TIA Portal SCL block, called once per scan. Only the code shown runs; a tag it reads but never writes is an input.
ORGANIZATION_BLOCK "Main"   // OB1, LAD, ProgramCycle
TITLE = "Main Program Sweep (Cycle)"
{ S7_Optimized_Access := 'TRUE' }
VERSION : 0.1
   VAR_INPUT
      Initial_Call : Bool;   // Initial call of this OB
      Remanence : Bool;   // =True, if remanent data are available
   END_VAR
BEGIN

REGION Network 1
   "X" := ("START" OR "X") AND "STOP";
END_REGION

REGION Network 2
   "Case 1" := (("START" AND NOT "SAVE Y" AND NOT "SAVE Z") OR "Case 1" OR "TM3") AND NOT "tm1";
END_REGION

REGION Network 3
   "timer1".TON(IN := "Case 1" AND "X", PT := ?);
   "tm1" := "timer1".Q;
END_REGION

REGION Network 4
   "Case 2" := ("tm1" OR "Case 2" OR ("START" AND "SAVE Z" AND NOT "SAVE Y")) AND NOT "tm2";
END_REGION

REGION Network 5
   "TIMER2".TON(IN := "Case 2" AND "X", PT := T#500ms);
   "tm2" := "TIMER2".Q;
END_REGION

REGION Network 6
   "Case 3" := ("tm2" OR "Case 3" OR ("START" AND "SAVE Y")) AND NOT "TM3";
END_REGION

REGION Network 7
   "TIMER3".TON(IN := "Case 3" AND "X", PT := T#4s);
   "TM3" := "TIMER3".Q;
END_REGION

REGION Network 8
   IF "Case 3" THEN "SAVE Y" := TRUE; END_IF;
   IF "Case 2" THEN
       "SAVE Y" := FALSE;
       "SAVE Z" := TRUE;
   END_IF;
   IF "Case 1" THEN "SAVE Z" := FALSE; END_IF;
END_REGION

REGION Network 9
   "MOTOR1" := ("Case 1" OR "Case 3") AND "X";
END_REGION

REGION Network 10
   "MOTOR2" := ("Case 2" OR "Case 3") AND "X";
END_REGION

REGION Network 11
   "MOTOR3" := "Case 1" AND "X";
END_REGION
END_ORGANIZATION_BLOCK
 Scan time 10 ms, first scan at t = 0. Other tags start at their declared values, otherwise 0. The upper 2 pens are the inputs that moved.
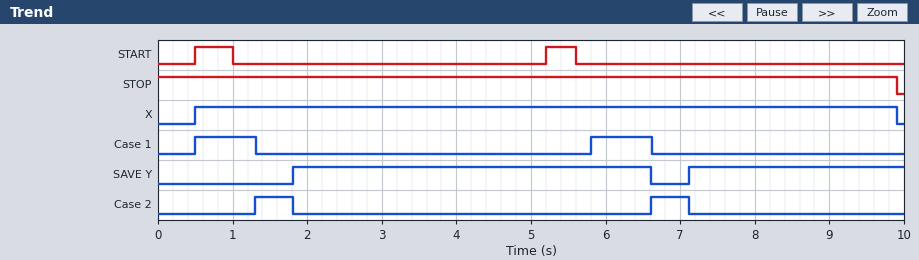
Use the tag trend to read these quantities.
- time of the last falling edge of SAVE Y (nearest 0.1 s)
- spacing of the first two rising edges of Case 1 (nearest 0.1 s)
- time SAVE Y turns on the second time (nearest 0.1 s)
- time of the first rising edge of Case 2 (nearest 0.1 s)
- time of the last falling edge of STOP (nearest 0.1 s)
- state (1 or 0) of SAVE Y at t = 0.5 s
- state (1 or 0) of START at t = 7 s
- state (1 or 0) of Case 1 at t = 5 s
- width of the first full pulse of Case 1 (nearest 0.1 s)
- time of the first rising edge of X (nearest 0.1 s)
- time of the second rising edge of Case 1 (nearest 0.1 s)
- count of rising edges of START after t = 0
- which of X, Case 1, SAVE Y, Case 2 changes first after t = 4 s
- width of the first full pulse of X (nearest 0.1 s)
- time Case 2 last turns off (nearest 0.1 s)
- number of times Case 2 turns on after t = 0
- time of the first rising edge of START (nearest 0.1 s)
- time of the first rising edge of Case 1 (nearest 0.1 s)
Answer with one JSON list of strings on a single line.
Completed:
["6.6 s", "5.3 s", "7.1 s", "1.3 s", "9.9 s", "0", "0", "0", "0.8 s", "0.5 s", "5.8 s", "2", "Case 1", "9.4 s", "7.1 s", "2", "0.5 s", "0.5 s"]
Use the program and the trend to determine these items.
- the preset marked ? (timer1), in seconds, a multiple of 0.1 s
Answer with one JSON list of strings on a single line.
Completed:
["0.8 s"]
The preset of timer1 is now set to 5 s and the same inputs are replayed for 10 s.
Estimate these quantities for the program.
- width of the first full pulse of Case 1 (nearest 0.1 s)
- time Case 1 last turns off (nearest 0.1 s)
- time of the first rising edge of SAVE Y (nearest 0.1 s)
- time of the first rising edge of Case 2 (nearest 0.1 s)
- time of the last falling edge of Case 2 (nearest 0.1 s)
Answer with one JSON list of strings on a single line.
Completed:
["5.0 s", "5.5 s", "6.0 s", "5.5 s", "6.0 s"]
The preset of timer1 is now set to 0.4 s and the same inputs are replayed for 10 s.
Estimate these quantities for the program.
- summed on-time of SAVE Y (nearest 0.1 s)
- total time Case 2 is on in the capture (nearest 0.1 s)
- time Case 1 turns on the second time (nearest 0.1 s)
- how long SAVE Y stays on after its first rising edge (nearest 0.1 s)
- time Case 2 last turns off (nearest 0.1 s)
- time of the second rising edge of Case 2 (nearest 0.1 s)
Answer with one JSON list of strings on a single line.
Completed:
["7.9 s", "1.2 s", "5.4 s", "4.4 s", "6.3 s", "5.8 s"]
